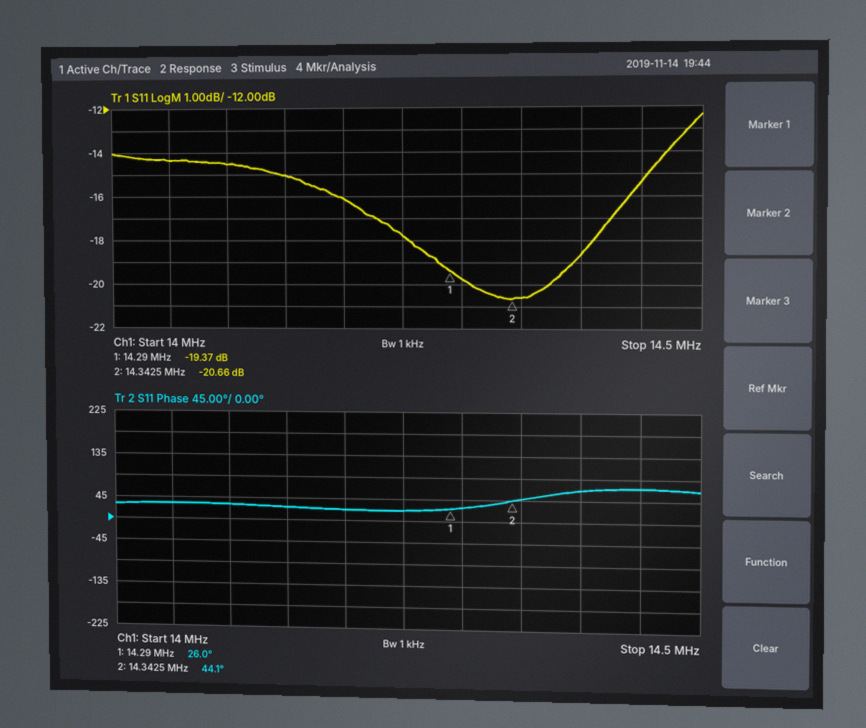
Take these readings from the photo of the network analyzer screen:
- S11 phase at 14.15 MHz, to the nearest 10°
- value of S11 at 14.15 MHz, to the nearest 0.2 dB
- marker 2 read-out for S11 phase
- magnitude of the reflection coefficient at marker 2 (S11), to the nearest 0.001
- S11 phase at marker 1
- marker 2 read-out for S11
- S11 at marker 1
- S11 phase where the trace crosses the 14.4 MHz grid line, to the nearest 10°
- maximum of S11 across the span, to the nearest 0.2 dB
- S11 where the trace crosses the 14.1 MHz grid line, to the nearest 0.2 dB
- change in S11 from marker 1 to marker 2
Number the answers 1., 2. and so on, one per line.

1. 30°
2. -15.0 dB
3. 44.1°
4. 0.093
5. 26.0°
6. -20.66 dB
7. -19.37 dB
8. 70°
9. -12.4 dB
10. -14.6 dB
11. -1.29 dB
